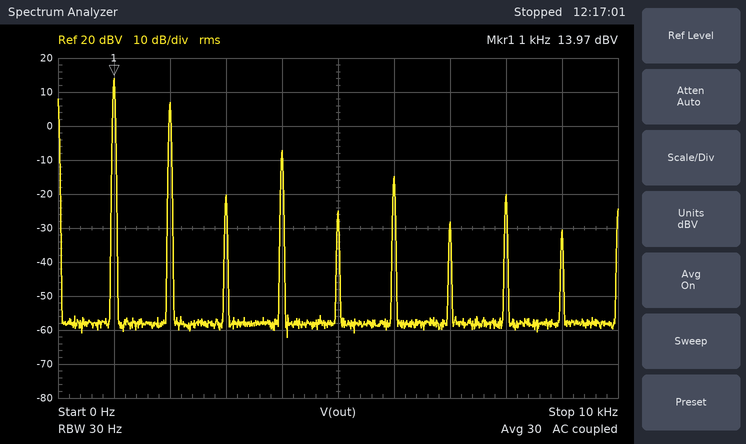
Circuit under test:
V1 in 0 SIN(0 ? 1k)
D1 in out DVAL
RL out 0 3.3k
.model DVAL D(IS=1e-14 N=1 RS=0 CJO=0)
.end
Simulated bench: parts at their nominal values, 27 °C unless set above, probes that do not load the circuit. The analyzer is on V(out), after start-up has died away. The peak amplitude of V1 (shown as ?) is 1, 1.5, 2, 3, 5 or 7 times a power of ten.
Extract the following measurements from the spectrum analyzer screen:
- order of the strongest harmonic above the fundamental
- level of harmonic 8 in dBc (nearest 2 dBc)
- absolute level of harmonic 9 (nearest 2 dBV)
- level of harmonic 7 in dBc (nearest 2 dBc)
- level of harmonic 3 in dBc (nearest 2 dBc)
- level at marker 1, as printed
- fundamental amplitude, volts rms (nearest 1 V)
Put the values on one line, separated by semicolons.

2; -34 dBc; -30 dBV; -42 dBc; -34 dBc; 13.97 dBV; 5 V
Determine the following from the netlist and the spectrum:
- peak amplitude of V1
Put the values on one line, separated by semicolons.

15 V
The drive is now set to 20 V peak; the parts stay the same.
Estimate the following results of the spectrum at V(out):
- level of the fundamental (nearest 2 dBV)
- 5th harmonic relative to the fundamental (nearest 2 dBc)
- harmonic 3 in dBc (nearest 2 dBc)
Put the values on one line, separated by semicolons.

16 dBV; -42 dBc; -36 dBc
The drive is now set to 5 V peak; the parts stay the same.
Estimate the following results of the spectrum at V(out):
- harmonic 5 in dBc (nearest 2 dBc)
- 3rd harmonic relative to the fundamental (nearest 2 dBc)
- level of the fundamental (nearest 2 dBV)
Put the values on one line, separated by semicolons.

-30 dBc; -24 dBc; 4 dBV
